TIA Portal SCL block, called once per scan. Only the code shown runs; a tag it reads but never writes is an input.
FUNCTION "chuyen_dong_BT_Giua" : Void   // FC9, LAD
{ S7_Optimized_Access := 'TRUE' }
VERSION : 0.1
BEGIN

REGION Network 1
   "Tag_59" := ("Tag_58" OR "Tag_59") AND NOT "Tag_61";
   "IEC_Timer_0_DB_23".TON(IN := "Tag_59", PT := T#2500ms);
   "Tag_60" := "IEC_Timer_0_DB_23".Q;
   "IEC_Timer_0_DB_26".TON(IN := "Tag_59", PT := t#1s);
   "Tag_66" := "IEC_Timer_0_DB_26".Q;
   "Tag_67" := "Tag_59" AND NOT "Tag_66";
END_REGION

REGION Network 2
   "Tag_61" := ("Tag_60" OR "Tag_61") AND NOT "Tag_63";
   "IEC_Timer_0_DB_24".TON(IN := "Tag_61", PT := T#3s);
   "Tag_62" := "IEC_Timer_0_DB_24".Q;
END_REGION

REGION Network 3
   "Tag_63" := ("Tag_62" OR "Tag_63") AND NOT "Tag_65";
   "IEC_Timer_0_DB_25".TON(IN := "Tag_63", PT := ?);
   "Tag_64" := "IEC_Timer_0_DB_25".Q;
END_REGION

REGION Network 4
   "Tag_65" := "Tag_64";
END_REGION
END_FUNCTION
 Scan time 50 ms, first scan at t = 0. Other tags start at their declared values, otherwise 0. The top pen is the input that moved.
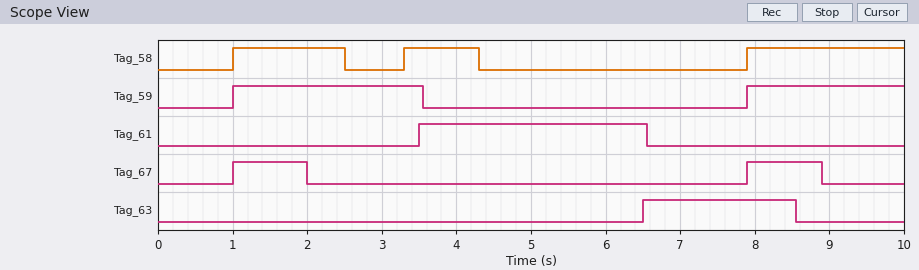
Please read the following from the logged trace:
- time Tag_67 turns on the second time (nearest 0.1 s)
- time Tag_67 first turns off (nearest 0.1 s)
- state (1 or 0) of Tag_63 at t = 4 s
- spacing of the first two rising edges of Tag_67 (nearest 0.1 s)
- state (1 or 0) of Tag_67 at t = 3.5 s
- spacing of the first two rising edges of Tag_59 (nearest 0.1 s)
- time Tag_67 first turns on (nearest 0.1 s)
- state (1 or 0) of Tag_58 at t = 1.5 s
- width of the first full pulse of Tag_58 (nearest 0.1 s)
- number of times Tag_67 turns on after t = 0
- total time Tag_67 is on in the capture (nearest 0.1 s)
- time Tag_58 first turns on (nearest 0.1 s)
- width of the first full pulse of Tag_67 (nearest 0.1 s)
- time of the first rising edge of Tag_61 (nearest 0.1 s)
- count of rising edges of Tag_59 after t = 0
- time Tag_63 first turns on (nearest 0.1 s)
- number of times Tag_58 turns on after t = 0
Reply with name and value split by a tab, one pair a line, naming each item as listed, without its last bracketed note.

time Tag_67 turns on the second time	7.9 s
time Tag_67 first turns off	2.0 s
state (1 or 0) of Tag_63 at t = 4 s	0
spacing of the first two rising edges of Tag_67	6.9 s
state (1 or 0) of Tag_67 at t = 3.5 s	0
spacing of the first two rising edges of Tag_59	6.9 s
time Tag_67 first turns on	1.0 s
state (1 or 0) of Tag_58 at t = 1.5 s	1
width of the first full pulse of Tag_58	1.5 s
number of times Tag_67 turns on after t = 0	2
total time Tag_67 is on in the capture	2.0 s
time Tag_58 first turns on	1.0 s
width of the first full pulse of Tag_67	1.0 s
time of the first rising edge of Tag_61	3.5 s
count of rising edges of Tag_59 after t = 0	2
time Tag_63 first turns on	6.5 s
number of times Tag_58 turns on after t = 0	3
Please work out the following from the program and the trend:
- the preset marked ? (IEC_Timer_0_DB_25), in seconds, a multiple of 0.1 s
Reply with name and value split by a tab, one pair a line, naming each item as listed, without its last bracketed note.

the preset marked ? (IEC_Timer_0_DB_25), in seconds, a multiple of 0.1 s	2.0 s
